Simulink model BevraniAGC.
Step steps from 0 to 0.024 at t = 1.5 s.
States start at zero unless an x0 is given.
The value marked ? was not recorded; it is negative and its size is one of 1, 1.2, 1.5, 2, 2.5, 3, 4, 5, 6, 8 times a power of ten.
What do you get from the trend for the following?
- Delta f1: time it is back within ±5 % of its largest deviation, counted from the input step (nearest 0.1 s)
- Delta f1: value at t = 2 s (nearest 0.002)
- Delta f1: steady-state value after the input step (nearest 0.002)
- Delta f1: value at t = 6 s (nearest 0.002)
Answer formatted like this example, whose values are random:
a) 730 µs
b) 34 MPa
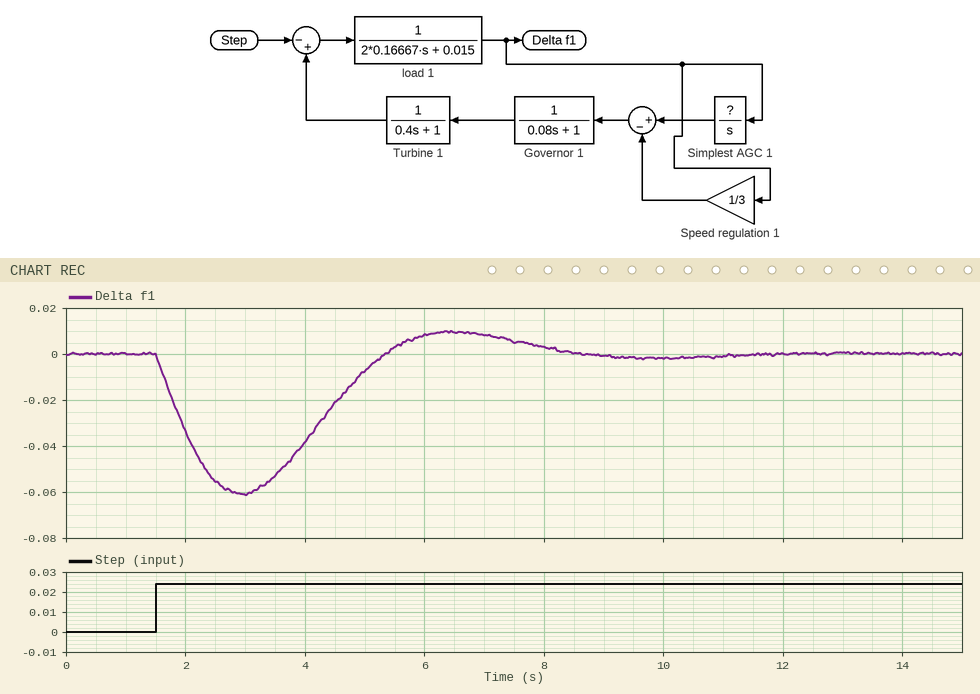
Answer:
a) 6.5 s
b) -0.034
c) 0.000
d) 0.008
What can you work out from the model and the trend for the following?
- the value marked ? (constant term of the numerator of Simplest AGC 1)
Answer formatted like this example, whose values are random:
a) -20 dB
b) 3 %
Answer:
a) -0.2
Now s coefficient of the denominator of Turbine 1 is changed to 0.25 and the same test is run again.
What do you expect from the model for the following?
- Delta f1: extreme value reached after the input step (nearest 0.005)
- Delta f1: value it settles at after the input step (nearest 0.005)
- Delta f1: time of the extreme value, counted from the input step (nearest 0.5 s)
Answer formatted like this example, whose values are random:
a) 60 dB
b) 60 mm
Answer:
a) -0.055
b) 0.000
c) 1.5 s
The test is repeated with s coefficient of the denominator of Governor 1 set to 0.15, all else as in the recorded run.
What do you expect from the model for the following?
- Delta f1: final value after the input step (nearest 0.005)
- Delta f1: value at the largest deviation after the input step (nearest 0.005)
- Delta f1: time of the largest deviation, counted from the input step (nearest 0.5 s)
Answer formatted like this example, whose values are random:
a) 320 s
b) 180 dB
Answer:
a) 0.000
b) -0.065
c) 1.5 s
